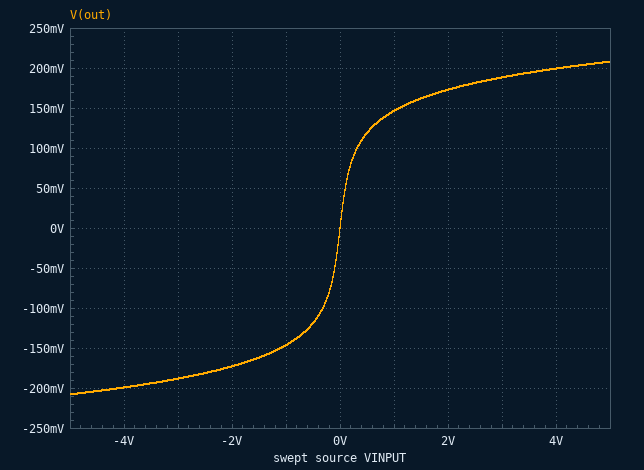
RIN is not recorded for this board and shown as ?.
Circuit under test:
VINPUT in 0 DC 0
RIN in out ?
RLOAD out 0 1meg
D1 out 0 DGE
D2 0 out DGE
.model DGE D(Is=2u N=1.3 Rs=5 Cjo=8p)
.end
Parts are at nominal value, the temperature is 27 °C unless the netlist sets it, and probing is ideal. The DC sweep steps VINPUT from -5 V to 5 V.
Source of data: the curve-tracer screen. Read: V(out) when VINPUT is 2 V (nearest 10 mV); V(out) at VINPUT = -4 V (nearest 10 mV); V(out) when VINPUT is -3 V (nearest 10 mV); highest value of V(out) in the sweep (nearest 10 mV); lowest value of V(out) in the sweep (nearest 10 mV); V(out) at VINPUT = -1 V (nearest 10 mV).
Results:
170 mV
-200 mV
-190 mV
210 mV
-210 mV
-150 mV
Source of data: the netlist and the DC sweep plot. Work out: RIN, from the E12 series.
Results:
5.6 kΩ
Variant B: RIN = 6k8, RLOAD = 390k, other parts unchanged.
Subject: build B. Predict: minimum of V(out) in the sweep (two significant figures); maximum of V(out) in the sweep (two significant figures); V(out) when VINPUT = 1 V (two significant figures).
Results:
-200 mV
200 mV
140 mV
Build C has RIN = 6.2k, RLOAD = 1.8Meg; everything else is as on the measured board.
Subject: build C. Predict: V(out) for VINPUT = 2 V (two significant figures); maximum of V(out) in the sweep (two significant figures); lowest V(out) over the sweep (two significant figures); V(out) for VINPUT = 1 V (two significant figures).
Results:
170 mV
200 mV
-200 mV
140 mV
